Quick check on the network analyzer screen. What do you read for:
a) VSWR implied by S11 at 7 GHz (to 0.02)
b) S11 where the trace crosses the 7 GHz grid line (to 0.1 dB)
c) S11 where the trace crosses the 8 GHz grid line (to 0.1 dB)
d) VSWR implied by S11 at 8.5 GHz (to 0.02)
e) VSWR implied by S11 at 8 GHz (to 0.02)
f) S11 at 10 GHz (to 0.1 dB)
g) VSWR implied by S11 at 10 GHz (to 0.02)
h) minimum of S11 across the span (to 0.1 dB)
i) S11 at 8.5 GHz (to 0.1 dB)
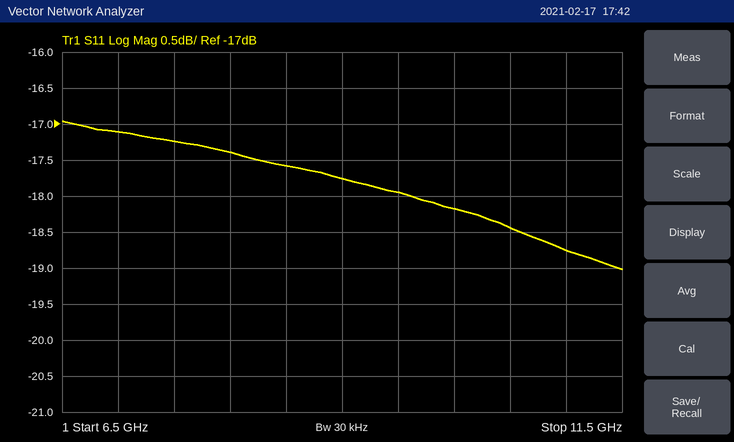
1.32
-17.1 dB
-17.4 dB
1.30
1.32
-18.2 dB
1.28
-19.0 dB
-17.6 dB
